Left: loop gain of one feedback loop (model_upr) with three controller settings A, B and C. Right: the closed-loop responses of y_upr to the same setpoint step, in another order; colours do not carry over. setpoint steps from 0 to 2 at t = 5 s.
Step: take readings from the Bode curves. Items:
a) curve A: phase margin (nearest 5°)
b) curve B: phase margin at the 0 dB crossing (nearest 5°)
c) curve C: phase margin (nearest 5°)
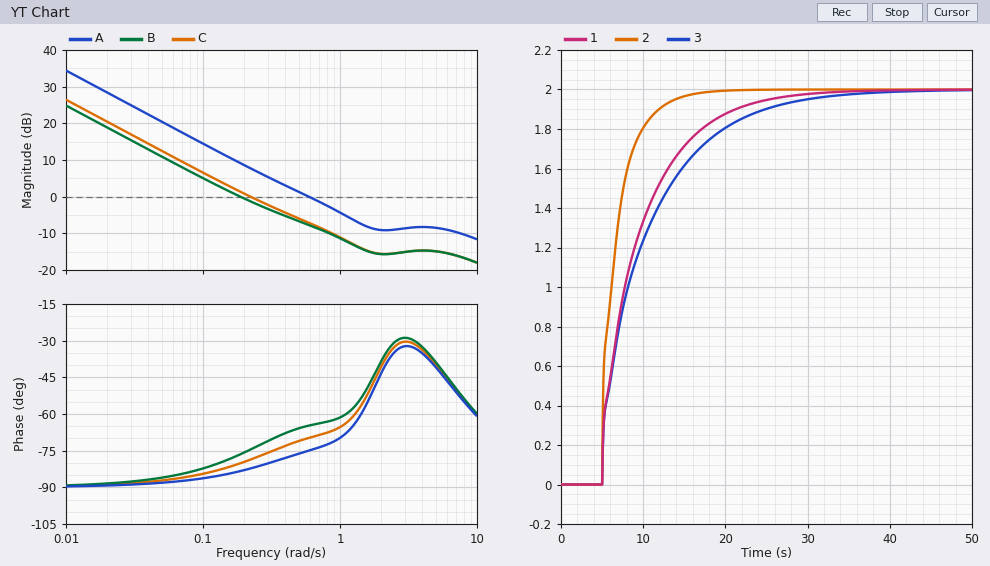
105°
105°
100°
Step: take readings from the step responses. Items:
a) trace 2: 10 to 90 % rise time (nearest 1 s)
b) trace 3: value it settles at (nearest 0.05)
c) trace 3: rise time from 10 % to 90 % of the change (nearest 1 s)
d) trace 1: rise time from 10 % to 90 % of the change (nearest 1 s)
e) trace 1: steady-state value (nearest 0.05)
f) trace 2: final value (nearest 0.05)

5 s
2.00
15 s
12 s
2.00
2.00
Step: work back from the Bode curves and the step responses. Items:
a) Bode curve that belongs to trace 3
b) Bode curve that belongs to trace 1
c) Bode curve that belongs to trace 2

B
C
A
